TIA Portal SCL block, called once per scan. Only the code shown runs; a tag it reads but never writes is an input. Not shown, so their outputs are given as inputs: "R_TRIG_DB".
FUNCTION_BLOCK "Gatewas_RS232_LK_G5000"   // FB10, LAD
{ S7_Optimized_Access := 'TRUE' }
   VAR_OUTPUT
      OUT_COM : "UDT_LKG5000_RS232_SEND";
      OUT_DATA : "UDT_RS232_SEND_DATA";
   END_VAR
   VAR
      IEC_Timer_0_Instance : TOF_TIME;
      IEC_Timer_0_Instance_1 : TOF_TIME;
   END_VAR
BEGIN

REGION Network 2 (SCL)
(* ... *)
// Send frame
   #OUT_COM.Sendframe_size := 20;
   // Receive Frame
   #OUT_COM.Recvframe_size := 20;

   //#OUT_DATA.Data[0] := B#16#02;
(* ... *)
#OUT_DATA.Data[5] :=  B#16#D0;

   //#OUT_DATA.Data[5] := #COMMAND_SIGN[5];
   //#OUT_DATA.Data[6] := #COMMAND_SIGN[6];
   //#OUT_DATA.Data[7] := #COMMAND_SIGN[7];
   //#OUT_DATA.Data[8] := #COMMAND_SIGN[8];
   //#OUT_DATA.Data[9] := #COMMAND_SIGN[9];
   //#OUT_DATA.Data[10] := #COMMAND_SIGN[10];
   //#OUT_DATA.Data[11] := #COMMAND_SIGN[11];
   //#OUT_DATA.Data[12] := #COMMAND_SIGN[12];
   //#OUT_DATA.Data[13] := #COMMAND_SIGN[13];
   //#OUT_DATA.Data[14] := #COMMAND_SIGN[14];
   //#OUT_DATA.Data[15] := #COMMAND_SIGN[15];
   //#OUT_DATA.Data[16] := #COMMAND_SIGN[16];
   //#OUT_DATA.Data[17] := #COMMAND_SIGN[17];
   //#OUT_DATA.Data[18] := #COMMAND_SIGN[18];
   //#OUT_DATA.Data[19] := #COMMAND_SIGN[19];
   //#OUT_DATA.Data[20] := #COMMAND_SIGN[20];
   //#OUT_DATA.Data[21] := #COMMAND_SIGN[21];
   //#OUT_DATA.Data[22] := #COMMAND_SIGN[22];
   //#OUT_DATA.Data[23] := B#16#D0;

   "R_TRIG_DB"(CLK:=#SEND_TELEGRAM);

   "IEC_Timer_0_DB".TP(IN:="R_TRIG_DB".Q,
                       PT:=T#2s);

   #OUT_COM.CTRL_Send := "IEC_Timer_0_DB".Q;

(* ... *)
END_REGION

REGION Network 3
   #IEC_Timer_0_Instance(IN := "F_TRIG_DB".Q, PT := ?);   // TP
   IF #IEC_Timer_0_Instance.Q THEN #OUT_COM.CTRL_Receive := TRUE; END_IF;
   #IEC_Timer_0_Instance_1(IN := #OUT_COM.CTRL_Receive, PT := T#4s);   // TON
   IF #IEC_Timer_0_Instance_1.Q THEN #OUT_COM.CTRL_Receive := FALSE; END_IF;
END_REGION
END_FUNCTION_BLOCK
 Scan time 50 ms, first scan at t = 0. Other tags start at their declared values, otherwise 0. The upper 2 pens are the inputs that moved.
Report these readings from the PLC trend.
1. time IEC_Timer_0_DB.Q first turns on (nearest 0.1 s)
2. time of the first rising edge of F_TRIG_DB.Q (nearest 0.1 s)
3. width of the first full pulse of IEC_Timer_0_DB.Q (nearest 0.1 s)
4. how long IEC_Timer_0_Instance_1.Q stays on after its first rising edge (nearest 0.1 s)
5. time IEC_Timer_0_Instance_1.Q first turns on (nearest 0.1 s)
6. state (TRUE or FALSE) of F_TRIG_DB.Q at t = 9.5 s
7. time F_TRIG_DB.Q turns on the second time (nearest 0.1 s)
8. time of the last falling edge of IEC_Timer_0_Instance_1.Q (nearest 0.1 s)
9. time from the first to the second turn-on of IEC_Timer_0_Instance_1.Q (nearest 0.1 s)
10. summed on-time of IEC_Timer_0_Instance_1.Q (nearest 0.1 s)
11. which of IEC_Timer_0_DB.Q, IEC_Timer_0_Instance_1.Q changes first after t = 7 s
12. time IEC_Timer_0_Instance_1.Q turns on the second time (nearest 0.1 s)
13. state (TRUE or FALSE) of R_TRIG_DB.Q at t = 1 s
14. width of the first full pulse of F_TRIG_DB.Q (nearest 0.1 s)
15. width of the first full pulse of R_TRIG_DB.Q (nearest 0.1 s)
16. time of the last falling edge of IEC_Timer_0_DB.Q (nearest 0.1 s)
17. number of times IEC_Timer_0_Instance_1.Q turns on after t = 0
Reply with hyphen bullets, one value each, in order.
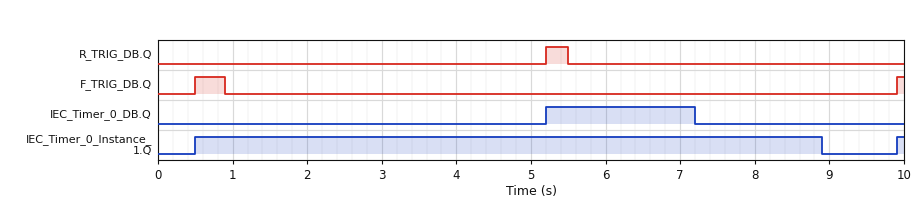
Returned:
- 5.2 s
- 0.5 s
- 2.0 s
- 8.4 s
- 0.5 s
- FALSE
- 9.9 s
- 8.9 s
- 9.4 s
- 8.5 s
- IEC_Timer_0_DB.Q
- 9.9 s
- FALSE
- 0.4 s
- 0.3 s
- 7.2 s
- 2
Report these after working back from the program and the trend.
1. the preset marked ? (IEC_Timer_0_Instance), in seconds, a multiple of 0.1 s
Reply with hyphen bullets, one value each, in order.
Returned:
- 4.0 s
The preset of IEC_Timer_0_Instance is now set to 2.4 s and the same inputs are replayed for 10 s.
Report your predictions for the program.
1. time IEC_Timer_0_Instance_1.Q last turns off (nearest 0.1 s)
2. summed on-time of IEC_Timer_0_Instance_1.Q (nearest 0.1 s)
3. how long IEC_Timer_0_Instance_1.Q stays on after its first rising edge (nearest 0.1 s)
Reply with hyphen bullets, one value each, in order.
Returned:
- 7.3 s
- 6.9 s
- 6.8 s
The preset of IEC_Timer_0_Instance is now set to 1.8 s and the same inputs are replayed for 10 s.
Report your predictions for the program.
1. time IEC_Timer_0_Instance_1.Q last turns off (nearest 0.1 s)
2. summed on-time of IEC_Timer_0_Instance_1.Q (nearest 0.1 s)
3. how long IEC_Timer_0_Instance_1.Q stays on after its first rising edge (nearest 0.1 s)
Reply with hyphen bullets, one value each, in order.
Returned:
- 6.7 s
- 6.3 s
- 6.2 s
